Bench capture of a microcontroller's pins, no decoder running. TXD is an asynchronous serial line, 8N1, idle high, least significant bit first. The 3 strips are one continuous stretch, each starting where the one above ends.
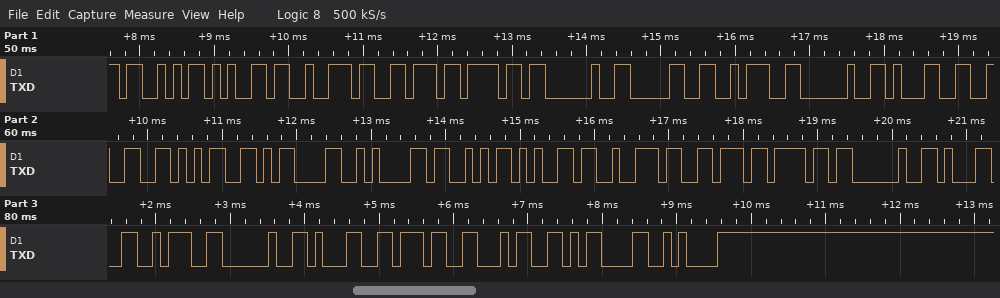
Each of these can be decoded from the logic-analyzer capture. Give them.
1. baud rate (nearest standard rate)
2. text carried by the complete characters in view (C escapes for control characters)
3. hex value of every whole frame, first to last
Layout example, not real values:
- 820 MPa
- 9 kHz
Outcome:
- 9600 baud
- "Servo 0: 125\r\nServo 1: 174\r\n"
- 0x53 0x65 0x72 0x76 0x6F 0x20 0x30 0x3A 0x20 0x31 0x32 0x35 0x0D 0x0A 0x53 0x65 0x72 0x76 0x6F 0x20 0x31 0x3A 0x20 0x31 0x37 0x34 0x0D 0x0A
